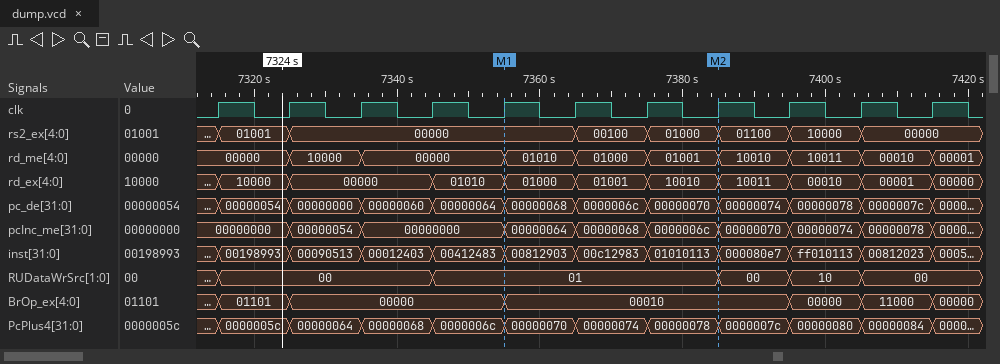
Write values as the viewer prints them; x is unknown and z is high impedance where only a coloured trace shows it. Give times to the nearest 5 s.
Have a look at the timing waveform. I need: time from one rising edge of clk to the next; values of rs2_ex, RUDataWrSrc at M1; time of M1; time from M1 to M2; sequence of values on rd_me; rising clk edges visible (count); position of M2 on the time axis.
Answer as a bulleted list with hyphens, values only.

- 10 s
- rs2_ex=00000, RUDataWrSrc=01
- 7355 s
- 30 s
- 00000, 10000, 00000, 01010, 01000, 01001, 10010, 10011, 00010, 00001
- 11
- 7385 s
